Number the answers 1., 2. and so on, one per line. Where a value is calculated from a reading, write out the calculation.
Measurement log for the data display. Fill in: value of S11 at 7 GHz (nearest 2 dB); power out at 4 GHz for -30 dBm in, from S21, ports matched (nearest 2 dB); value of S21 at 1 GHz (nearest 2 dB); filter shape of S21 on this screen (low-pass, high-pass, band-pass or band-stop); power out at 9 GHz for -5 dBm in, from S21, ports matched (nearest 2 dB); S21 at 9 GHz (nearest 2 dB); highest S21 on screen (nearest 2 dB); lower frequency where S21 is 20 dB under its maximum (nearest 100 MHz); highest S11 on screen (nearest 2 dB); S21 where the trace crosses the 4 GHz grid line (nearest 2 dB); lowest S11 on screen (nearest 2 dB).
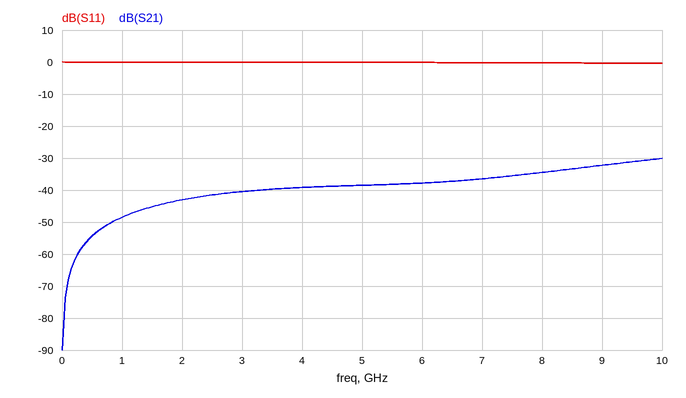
1. 0 dB
2. -30 dBm + (-40 dB) = -70 dBm
3. -48 dB
4. high-pass
5. -5 dBm + (-32 dB) = -38 dBm
6. -32 dB
7. -30 dB
8. 800 MHz
9. 0 dB
10. -40 dB
11. 0 dB
